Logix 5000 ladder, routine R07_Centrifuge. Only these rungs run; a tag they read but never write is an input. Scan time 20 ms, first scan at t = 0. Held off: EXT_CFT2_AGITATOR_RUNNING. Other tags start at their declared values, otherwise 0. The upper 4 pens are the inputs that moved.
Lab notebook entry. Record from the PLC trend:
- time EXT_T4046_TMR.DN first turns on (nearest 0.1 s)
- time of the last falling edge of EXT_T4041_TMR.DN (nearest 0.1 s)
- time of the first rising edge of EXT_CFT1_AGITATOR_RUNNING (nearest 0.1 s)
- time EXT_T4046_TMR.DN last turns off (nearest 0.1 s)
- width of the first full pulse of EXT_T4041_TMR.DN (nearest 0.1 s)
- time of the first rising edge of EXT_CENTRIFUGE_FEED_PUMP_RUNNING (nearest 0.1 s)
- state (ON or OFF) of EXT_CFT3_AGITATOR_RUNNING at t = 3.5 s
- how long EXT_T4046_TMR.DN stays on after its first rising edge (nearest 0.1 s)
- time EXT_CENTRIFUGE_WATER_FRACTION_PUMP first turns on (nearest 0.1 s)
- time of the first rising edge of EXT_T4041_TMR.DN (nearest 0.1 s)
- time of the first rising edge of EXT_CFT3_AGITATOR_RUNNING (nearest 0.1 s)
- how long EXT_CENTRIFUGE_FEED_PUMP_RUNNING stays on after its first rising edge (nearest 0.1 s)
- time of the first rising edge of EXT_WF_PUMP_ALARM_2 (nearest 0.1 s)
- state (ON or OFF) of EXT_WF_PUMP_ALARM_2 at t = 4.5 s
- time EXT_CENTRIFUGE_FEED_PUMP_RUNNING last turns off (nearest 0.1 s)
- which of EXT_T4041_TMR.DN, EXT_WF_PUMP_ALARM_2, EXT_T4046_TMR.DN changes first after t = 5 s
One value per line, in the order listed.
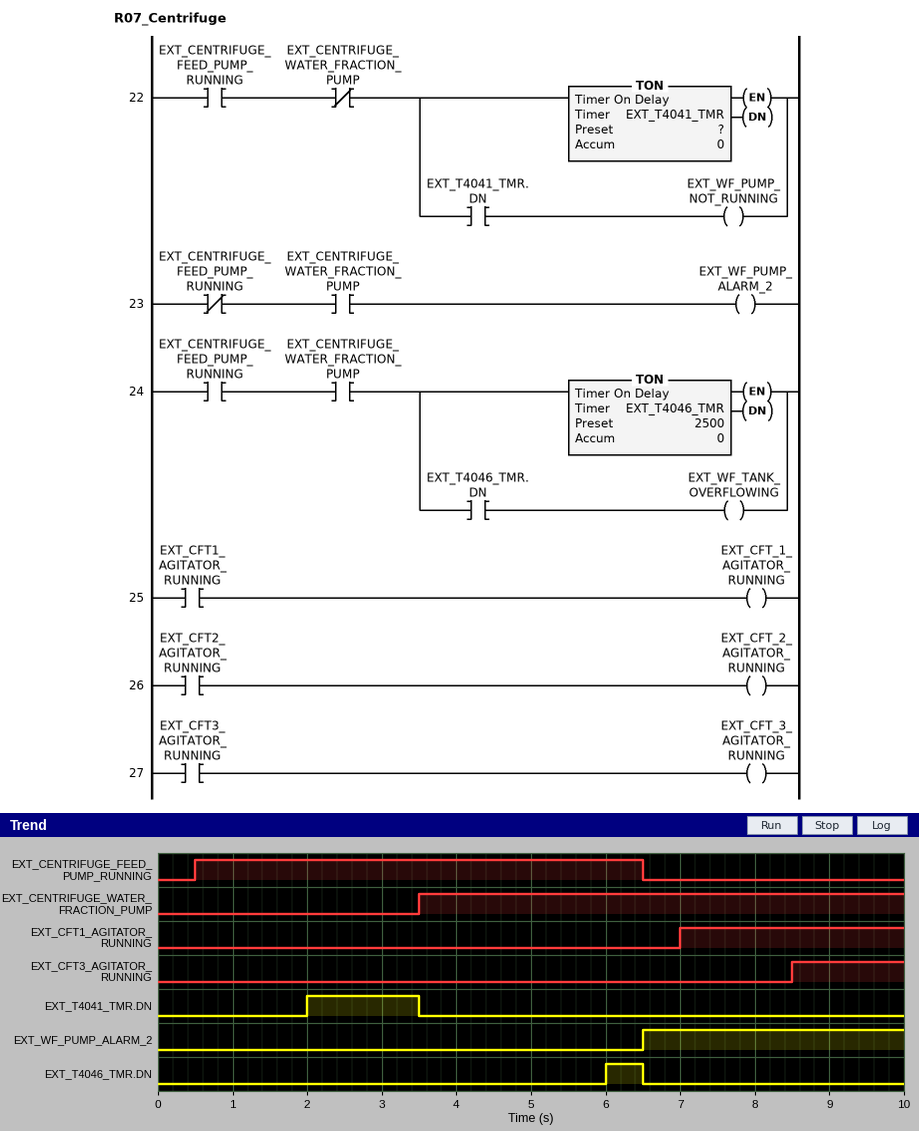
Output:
6.0 s
3.5 s
7.0 s
6.5 s
1.5 s
0.5 s
OFF
0.5 s
3.5 s
2.0 s
8.5 s
6.0 s
6.5 s
OFF
6.5 s
EXT_T4046_TMR.DN
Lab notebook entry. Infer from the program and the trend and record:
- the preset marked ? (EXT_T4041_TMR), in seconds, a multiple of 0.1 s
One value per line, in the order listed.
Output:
1.5 s
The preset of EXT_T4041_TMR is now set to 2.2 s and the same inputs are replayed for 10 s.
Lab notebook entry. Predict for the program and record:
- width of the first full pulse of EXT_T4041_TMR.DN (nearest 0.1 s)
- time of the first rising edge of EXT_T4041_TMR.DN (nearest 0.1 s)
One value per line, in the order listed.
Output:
0.8 s
2.7 s
